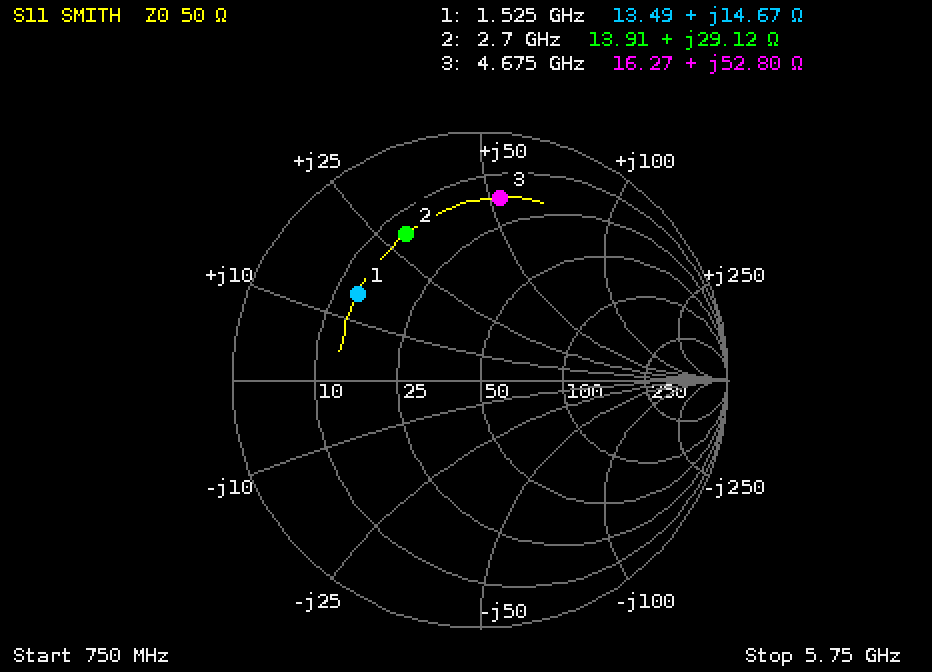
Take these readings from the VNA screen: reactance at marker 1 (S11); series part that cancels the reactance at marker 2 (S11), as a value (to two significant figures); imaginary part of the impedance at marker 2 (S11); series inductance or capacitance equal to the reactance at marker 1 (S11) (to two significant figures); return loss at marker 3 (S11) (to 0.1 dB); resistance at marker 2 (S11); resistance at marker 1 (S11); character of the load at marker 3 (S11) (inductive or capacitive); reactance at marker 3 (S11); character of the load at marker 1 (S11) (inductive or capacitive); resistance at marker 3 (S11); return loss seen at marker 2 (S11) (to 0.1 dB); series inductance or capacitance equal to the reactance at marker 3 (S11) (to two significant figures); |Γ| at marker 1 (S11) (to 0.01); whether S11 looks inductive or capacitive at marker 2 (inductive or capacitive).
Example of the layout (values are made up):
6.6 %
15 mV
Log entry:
+14.67 Ω
2.0 pF
+29.12 Ω
1.5 nH
2.6 dB
13.91 Ω
13.49 Ω
inductive
+52.80 Ω
inductive
16.27 Ω
3.6 dB
1.8 nH
0.60
inductive
